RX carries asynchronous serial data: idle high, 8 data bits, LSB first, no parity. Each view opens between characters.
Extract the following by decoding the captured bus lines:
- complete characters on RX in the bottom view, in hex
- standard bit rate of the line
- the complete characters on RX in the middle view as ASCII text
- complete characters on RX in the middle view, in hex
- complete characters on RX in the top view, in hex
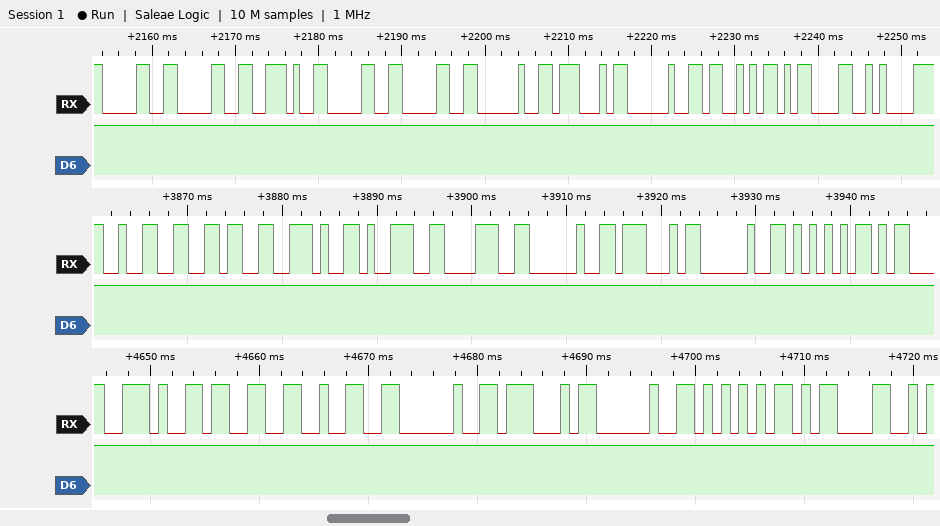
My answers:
2E, 33, 32, 20, 47, 20, 55, 0D
1200 baud
"26.98 G U"
32, 36, 2E, 39, 38, 20, 47, 20, 55
30, 30, 2E, 30, 30, 20, 47, 20, 53, 0D, 0A
